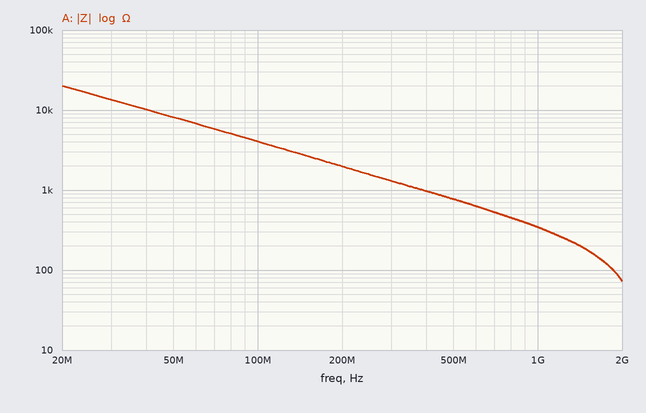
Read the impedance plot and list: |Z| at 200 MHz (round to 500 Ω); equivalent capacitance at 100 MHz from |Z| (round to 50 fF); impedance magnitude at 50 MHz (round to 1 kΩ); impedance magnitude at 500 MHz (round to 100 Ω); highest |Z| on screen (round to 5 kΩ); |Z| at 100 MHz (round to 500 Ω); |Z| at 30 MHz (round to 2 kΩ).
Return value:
2.0 kΩ
400 fF
8 kΩ
800 Ω
20 kΩ
4.0 kΩ
14 kΩ
